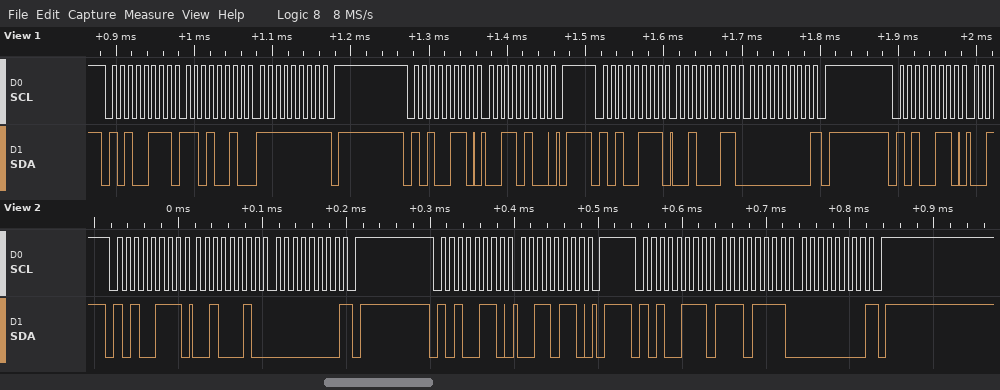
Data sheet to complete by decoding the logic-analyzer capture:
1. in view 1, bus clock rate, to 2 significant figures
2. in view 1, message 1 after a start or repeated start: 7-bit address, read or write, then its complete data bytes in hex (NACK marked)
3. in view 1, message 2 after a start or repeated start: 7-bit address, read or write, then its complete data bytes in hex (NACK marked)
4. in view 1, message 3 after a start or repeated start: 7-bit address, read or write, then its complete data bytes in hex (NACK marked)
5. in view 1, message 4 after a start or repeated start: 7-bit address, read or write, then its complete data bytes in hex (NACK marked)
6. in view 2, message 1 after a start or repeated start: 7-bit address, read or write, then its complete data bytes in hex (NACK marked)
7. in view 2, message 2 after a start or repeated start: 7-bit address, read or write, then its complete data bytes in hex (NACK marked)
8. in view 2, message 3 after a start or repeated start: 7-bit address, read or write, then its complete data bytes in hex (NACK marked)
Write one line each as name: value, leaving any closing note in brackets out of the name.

in view 1, bus clock rate, to 2 significant figures: 100 kHz
in view 1, message 1 after a start or repeated start: 7-bit address, read or write, then its complete data bytes in hex: 0x53 read: D2 FF NACK
in view 1, message 2 after a start or repeated start: 7-bit address, read or write, then its complete data bytes in hex: 0x53 write: 34
in view 1, message 3 after a start or repeated start: 7-bit address, read or write, then its complete data bytes in hex: 0x53 read: 23 00 NACK
in view 1, message 4 after a start or repeated start: 7-bit address, read or write, then its complete data bytes in hex: 0x53 write
in view 2, message 1 after a start or repeated start: 7-bit address, read or write, then its complete data bytes in hex: 0x53 read: 22 00 NACK
in view 2, message 2 after a start or repeated start: 7-bit address, read or write, then its complete data bytes in hex: 0x53 write: 36
in view 2, message 3 after a start or repeated start: 7-bit address, read or write, then its complete data bytes in hex: 0x53 read: EF 00 NACK
